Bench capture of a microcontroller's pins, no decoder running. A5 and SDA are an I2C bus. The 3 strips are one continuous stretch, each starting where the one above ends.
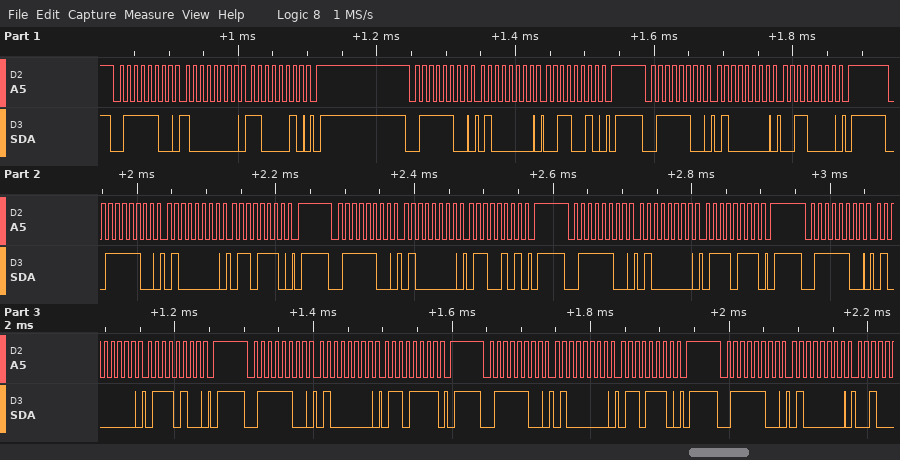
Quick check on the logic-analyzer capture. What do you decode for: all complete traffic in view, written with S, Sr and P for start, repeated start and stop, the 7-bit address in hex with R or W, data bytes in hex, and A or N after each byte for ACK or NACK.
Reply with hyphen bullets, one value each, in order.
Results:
- S 3EW A 80 A C2 A P S 3EW A 40 A 32 A P S 3EW A 40 A 30 A P S 3EW A 40 A 6E A P S 3EW A 40 A 65 A P S 3EW A 40 A 77 A P S 3EW A 40 A 74 A P S 3EW A 40 A 6F A P S 3EW A 40 A 6E A P S 3EW A 40 A
